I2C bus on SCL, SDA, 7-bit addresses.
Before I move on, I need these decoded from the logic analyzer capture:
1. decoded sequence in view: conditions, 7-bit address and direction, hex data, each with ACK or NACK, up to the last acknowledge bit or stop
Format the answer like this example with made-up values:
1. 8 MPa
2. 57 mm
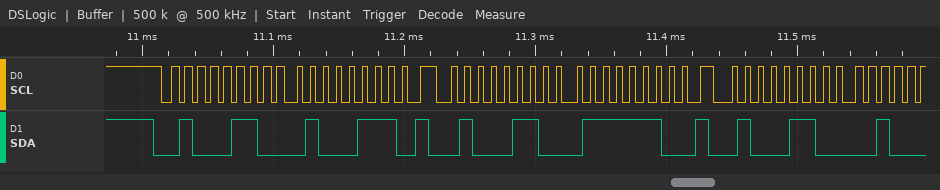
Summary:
1. start, address 23 write ACK, 47 ACK, repeated start, address 23 write ACK, 7E ACK, repeated start, address 23 write ACK
